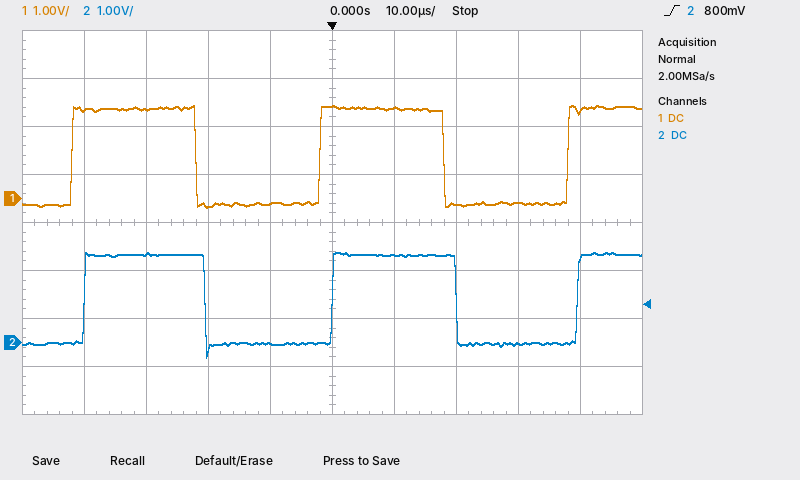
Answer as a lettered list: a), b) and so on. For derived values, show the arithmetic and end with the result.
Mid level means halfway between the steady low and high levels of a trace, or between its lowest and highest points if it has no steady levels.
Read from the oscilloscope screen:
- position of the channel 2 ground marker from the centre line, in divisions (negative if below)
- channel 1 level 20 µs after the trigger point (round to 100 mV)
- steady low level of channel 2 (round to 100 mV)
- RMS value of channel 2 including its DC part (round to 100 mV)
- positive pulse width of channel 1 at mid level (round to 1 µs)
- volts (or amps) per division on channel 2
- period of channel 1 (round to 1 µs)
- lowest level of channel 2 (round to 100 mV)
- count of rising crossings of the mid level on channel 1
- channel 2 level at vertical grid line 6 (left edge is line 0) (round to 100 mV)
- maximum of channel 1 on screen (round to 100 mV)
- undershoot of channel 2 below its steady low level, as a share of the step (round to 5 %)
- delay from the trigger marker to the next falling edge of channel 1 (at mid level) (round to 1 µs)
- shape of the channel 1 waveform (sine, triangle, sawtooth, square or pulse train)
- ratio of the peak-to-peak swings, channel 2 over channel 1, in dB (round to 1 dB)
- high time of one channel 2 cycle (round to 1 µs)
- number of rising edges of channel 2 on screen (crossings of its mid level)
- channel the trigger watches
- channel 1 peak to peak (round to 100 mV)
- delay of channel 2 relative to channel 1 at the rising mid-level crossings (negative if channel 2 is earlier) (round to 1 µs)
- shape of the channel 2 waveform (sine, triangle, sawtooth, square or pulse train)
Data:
a) -2.5 div
b) -100 mV
c) 0.0 V
d) √(0.5 × (1.9 V)² + 0.5 × (0.0 V)²) ≈ 1.3 V
e) 20 µs
f) 1 V
g) 40 µs
h) -300 mV
i) 3
j) 1.8 V
k) 1.9 V
l) 15 %
m) 18 µs
n) square
o) 20 log10(2.2 V / 2.1 V) ≈ 0 dB
p) 20 µs
q) 3
r) channel 2
s) 1.9 V − (-200 mV) = 2.1 V
t) +2 µs
u) square
